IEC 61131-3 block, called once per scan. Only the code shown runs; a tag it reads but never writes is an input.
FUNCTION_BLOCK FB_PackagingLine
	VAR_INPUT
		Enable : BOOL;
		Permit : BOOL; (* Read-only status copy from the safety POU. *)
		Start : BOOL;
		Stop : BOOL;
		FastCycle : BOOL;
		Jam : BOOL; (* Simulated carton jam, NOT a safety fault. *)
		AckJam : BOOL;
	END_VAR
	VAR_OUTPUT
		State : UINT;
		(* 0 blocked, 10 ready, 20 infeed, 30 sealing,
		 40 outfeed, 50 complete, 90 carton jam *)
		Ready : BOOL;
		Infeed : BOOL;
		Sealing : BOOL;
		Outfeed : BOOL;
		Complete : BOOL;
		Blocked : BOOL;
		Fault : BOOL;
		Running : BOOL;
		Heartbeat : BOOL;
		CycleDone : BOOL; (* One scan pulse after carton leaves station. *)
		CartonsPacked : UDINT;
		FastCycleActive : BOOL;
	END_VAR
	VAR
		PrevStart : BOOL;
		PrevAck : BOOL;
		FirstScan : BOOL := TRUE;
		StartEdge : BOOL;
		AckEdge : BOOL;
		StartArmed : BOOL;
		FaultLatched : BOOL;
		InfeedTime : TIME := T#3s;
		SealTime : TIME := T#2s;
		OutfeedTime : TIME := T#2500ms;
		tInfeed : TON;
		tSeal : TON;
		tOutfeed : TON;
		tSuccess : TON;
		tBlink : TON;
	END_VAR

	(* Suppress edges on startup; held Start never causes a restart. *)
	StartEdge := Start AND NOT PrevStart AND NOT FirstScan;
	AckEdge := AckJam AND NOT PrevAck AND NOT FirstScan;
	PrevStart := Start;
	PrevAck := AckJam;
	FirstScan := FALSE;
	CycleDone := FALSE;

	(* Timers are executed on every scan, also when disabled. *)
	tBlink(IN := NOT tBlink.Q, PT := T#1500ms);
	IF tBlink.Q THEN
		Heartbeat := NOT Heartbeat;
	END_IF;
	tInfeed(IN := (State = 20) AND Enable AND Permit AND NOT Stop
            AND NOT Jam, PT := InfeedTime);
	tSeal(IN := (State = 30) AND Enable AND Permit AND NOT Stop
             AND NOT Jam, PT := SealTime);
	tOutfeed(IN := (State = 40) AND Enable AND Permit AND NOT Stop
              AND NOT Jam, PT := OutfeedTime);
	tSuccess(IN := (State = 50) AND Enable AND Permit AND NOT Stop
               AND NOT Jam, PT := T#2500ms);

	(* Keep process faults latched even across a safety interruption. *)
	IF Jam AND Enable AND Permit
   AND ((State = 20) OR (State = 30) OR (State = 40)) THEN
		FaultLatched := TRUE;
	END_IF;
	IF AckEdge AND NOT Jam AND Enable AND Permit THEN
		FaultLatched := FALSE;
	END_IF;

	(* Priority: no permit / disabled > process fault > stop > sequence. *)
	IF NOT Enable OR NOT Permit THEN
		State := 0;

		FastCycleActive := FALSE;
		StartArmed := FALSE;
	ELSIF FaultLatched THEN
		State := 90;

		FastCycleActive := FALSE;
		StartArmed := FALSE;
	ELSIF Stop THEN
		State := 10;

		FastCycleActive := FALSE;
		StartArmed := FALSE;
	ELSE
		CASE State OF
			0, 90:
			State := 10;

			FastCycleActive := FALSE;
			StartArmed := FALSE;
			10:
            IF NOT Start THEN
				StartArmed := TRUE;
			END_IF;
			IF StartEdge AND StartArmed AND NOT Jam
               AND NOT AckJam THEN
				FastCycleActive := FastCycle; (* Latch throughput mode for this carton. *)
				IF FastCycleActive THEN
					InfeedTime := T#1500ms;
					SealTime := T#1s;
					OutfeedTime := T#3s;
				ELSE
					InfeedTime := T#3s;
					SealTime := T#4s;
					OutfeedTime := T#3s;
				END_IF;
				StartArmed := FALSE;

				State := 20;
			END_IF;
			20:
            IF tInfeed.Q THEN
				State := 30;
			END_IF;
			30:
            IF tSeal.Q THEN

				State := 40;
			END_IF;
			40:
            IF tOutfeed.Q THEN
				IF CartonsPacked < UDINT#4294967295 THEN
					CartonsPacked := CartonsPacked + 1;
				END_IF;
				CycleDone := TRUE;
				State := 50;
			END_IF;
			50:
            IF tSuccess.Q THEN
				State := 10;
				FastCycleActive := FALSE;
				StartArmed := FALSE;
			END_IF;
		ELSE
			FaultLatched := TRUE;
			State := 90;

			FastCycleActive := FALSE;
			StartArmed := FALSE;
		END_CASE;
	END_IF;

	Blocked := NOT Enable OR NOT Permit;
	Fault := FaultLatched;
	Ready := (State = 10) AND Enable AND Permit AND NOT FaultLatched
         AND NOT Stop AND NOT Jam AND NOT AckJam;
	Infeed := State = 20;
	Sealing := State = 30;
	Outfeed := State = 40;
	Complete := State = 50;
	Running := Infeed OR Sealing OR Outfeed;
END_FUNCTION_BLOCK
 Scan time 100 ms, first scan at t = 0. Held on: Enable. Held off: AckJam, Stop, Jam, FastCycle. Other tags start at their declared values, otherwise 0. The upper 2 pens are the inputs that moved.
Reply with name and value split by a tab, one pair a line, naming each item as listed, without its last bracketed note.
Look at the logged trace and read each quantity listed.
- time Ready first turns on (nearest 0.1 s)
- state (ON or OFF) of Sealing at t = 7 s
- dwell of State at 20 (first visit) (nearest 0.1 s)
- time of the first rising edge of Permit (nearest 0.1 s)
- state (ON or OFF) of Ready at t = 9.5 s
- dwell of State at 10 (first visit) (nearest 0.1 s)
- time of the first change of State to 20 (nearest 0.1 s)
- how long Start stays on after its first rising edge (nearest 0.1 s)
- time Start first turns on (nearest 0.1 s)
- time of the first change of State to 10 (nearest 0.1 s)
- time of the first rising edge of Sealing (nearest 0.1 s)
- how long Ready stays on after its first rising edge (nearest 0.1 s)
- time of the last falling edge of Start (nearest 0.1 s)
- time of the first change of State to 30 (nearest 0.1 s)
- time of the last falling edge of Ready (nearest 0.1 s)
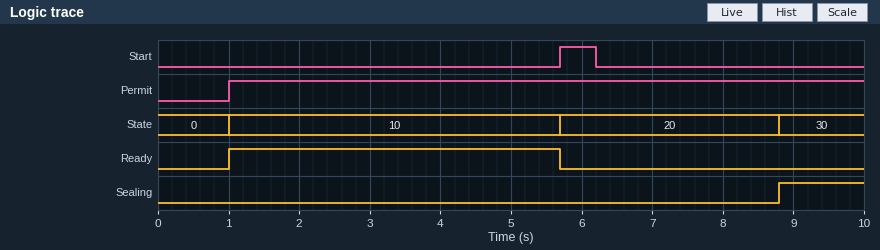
time Ready first turns on	1.0 s
state (ON or OFF) of Sealing at t = 7 s	OFF
dwell of State at 20 (first visit)	3.1 s
time of the first rising edge of Permit	1.0 s
state (ON or OFF) of Ready at t = 9.5 s	OFF
dwell of State at 10 (first visit)	4.7 s
time of the first change of State to 20	5.7 s
how long Start stays on after its first rising edge	0.5 s
time Start first turns on	5.7 s
time of the first change of State to 10	1.0 s
time of the first rising edge of Sealing	8.8 s
how long Ready stays on after its first rising edge	4.7 s
time of the last falling edge of Start	6.2 s
time of the first change of State to 30	8.8 s
time of the last falling edge of Ready	5.7 s
